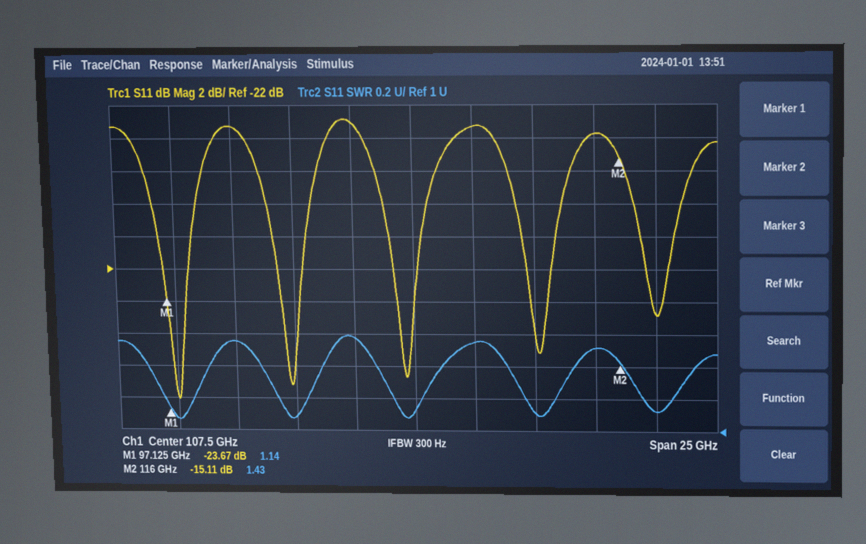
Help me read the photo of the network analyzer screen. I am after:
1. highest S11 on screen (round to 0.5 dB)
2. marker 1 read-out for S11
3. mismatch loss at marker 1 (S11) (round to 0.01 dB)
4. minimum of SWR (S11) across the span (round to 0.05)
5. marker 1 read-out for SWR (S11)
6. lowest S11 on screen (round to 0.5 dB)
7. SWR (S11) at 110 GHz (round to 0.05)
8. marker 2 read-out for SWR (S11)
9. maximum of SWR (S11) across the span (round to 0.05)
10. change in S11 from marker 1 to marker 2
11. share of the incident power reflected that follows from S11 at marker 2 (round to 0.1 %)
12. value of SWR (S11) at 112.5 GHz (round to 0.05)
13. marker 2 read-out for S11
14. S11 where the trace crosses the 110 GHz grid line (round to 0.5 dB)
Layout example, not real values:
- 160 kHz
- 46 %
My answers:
- -13.0 dB
- -23.67 dB
- 0.02 dB
- 1.05
- 1.14
- -30.0 dB
- 1.55
- 1.43
- 1.60
- 8.56 dB
- 3.1 %
- 1.10
- -15.11 dB
- -13.5 dB
